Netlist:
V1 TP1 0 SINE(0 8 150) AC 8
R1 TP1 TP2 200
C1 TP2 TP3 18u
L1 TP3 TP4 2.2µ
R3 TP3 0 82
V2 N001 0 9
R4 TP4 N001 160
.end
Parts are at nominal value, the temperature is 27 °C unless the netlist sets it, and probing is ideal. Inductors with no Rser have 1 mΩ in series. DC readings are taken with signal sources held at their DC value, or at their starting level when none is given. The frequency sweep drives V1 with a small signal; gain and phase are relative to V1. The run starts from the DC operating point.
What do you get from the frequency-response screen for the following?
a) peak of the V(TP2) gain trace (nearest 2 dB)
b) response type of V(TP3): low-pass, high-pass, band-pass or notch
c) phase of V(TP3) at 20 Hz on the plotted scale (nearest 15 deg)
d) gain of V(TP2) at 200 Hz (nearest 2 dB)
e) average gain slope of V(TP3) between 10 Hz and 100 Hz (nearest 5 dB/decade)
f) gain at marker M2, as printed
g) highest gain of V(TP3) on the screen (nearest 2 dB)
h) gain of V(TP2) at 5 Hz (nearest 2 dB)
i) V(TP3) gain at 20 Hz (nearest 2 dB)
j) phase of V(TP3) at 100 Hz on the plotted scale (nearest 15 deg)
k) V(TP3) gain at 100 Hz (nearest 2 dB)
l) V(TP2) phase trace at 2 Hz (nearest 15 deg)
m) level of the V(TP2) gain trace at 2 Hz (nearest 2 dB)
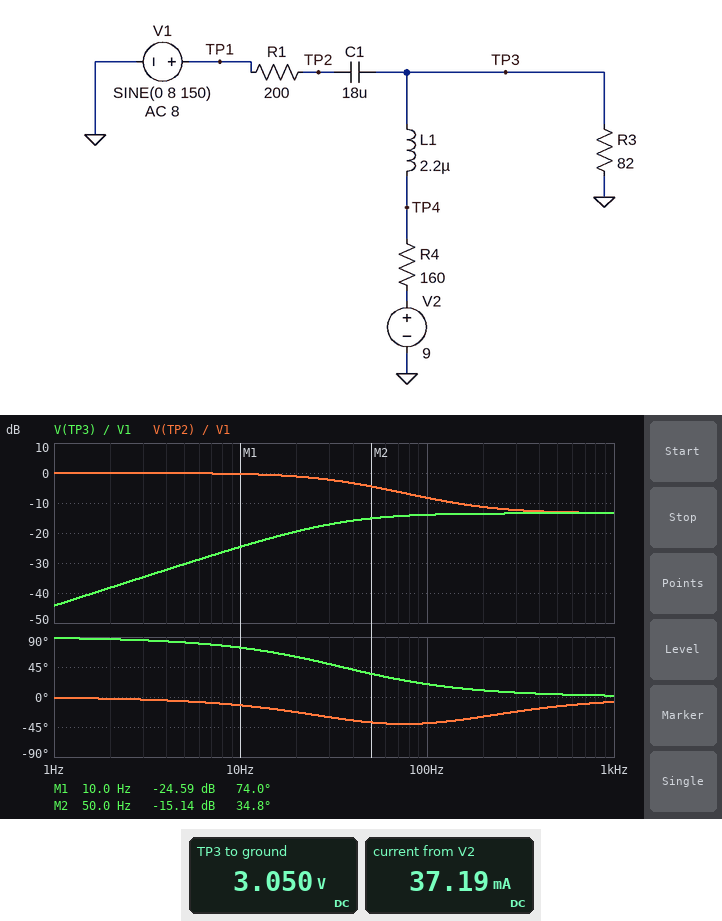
0 dB
high-pass
60 deg
-12 dB
10 dB/decade
-15.14 dB
-14 dB
0 dB
-20 dB
15 deg
-14 dB
0 deg
0 dB
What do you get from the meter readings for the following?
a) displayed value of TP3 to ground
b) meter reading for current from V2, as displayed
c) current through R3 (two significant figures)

3.050 V
37.19 mA
37 mA
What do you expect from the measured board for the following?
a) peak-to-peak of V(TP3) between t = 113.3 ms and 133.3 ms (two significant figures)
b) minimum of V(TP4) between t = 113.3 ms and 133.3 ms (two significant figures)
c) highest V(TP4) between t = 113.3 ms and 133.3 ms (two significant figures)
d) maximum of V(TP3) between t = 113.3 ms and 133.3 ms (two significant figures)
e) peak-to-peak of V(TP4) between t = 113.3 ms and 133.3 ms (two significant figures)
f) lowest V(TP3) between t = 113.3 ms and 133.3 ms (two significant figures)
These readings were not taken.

3.3 V
1.4 V
4.7 V
4.7 V
3.3 V
1.4 V
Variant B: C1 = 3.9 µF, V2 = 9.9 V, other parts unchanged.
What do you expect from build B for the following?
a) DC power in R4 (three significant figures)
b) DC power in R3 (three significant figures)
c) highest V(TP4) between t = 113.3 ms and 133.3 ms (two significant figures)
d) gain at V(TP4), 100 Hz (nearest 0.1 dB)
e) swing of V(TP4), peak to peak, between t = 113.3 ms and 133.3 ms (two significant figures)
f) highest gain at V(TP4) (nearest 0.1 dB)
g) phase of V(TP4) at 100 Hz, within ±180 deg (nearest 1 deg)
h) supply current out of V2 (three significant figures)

268 mW
137 mW
4.5 V
-19.0 dB
2.3 V
-13.4 dB
58 deg
40.9 mA
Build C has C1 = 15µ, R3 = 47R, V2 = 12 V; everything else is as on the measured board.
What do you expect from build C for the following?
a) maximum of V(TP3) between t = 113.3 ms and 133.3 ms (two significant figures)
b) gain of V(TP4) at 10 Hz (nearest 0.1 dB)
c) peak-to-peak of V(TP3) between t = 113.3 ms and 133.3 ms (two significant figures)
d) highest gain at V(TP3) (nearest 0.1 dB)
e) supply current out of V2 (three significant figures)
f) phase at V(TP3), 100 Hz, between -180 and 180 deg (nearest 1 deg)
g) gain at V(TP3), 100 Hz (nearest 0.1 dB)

3.9 V
-29.5 dB
2.4 V
-16.3 dB
58.0 mA
24 deg
-17.1 dB
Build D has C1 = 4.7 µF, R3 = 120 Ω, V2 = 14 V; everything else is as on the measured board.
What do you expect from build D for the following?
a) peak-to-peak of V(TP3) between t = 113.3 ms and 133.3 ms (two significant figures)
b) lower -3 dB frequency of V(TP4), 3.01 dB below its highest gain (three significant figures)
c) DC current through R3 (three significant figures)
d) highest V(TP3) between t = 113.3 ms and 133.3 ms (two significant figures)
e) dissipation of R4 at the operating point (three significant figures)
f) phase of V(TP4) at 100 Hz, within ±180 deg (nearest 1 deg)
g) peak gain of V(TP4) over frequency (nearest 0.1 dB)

3.1 V
126 Hz
50.0 mA
7.6 V
400 mW
52 deg
-11.9 dB
